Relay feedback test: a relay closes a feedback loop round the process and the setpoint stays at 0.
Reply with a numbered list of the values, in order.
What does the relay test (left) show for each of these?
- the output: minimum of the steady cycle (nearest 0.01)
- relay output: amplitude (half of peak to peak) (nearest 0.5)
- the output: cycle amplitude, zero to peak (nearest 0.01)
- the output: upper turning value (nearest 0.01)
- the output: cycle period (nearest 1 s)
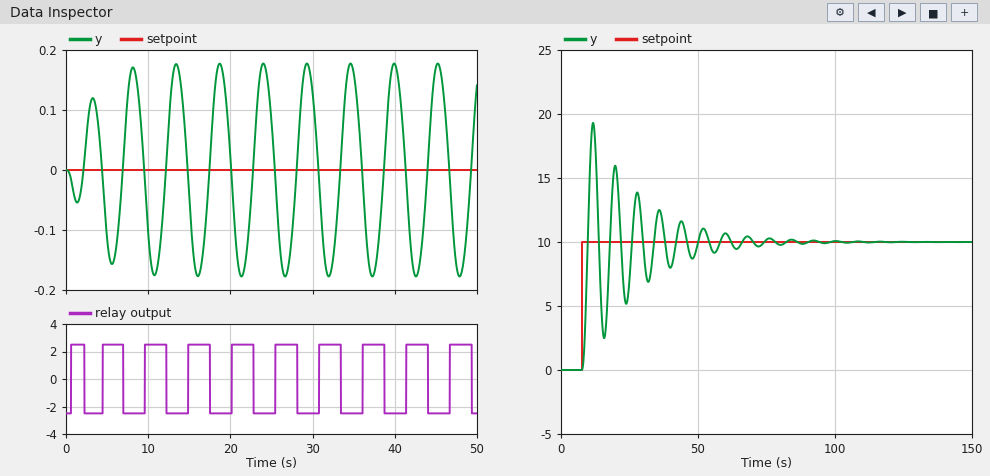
1. -0.18
2. 2.5
3. 0.18
4. 0.18
5. 5 s
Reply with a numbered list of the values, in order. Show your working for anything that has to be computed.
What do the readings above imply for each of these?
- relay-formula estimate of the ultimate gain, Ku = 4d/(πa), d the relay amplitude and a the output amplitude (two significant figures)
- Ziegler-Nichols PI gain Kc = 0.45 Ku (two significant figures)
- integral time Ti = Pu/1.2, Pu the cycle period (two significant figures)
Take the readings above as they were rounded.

1. 4 × 2.5 / (π × 0.18) = 18
2. 0.45 × 18 = 8.1
3. 5 / 1.2 = 4.2 s
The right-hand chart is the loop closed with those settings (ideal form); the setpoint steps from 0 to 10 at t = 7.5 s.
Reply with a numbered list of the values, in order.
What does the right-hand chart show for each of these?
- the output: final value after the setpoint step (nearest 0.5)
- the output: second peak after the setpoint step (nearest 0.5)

1. 10.0
2. 16.0
